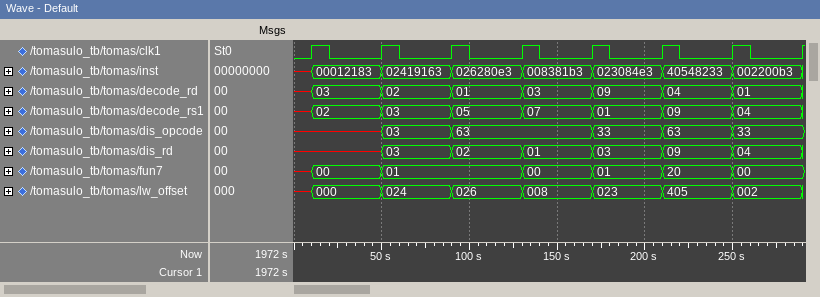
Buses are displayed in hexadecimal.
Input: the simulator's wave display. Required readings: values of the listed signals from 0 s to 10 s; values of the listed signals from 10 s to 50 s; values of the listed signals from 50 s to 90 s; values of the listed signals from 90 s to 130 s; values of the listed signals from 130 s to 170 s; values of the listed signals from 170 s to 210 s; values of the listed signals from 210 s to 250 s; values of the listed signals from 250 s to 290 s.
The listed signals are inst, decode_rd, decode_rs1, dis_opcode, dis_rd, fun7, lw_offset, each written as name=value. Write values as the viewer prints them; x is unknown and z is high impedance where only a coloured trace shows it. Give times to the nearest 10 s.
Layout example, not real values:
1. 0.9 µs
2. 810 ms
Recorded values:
1. inst=x, decode_rd=x, decode_rs1=x, dis_opcode=x, dis_rd=x, fun7=x, lw_offset=x
2. inst=00012183, decode_rd=03, decode_rs1=02, dis_opcode=x, dis_rd=x, fun7=00, lw_offset=000
3. inst=02419163, decode_rd=02, decode_rs1=03, dis_opcode=03, dis_rd=03, fun7=01, lw_offset=024
4. inst=026280e3, decode_rd=01, decode_rs1=05, dis_opcode=63, dis_rd=02, fun7=01, lw_offset=026
5. inst=008381b3, decode_rd=03, decode_rs1=07, dis_opcode=63, dis_rd=01, fun7=00, lw_offset=008
6. inst=023084e3, decode_rd=09, decode_rs1=01, dis_opcode=33, dis_rd=03, fun7=01, lw_offset=023
7. inst=40548233, decode_rd=04, decode_rs1=09, dis_opcode=63, dis_rd=09, fun7=20, lw_offset=405
8. inst=002200b3, decode_rd=01, decode_rs1=04, dis_opcode=33, dis_rd=04, fun7=00, lw_offset=002
